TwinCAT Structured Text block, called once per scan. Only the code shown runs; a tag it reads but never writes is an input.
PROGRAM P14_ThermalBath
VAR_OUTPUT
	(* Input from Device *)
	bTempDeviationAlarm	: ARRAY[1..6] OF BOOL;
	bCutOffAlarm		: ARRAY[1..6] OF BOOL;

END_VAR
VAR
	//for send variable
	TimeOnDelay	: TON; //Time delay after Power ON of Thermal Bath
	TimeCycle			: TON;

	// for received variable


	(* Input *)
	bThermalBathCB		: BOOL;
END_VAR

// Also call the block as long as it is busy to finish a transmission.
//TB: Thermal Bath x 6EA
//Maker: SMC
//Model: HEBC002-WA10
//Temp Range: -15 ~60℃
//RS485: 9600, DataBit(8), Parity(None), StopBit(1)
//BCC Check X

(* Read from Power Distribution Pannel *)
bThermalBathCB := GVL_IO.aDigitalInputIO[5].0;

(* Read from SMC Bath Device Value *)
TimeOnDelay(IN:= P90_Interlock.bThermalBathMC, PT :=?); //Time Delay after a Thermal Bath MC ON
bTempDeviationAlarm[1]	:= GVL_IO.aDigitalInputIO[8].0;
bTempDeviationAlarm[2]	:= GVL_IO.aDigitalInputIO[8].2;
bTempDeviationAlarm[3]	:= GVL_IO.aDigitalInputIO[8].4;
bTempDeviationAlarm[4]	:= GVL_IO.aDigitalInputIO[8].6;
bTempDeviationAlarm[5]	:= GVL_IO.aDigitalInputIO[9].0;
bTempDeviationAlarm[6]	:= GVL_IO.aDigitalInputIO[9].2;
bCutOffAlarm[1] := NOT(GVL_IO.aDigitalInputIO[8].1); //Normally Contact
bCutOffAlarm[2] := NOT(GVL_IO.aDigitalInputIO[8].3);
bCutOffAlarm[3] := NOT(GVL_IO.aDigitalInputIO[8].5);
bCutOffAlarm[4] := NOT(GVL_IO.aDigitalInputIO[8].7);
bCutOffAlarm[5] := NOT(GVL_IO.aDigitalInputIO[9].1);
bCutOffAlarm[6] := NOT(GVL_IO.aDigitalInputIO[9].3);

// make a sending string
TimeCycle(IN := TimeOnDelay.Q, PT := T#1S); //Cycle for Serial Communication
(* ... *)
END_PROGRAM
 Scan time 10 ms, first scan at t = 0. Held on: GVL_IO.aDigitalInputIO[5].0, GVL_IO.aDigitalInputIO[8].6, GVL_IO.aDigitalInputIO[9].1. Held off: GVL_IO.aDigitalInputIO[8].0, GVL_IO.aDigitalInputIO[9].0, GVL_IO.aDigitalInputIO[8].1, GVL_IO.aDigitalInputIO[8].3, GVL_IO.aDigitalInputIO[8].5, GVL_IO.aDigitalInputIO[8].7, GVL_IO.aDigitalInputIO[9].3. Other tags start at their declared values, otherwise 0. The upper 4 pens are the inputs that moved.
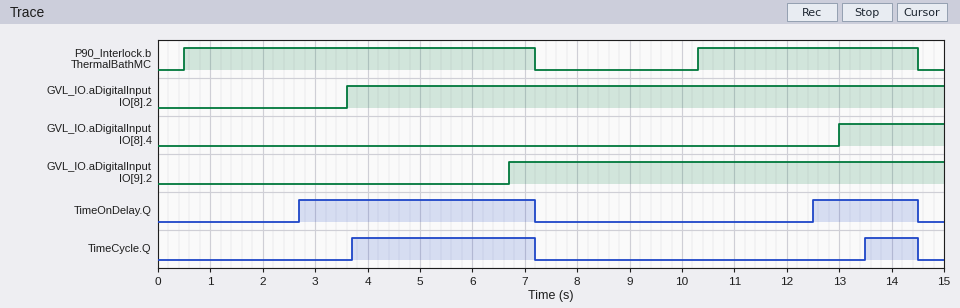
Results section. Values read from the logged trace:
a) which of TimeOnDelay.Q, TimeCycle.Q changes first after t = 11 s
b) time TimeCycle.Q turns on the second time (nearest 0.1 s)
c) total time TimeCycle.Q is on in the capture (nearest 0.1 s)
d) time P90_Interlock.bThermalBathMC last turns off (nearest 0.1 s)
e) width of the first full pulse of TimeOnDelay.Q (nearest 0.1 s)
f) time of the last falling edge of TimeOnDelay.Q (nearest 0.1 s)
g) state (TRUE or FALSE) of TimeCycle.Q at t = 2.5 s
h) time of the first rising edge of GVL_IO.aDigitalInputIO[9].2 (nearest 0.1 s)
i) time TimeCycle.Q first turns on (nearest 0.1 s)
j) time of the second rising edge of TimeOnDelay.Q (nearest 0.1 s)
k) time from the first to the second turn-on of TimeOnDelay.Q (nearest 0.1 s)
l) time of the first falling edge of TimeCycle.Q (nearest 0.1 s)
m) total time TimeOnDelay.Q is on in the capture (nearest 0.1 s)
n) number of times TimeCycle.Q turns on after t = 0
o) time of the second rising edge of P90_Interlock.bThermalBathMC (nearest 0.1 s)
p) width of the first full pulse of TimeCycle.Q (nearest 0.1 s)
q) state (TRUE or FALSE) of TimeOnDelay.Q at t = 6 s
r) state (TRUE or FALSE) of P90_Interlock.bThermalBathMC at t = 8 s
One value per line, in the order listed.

TimeOnDelay.Q
13.5 s
4.5 s
14.5 s
4.5 s
14.5 s
FALSE
6.7 s
3.7 s
12.5 s
9.8 s
7.2 s
6.5 s
2
10.3 s
3.5 s
TRUE
FALSE
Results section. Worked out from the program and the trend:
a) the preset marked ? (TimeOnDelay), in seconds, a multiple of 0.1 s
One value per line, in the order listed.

2.2 s
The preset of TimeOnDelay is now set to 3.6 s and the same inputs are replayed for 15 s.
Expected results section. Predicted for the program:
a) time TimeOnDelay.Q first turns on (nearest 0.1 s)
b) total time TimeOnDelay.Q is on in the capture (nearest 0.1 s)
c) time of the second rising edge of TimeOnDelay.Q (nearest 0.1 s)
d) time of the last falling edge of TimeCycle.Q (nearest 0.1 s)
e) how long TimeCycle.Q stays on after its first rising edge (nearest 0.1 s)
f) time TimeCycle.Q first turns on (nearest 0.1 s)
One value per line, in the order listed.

4.1 s
3.7 s
13.9 s
7.2 s
2.1 s
5.1 s
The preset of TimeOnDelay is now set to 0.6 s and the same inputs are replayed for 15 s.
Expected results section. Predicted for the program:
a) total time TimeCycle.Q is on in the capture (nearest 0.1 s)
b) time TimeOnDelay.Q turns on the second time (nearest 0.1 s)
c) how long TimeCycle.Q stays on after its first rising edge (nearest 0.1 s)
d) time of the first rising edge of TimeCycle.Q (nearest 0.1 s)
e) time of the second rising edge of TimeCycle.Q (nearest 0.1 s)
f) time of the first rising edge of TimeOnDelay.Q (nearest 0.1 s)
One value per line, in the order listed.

7.7 s
10.9 s
5.1 s
2.1 s
11.9 s
1.1 s
